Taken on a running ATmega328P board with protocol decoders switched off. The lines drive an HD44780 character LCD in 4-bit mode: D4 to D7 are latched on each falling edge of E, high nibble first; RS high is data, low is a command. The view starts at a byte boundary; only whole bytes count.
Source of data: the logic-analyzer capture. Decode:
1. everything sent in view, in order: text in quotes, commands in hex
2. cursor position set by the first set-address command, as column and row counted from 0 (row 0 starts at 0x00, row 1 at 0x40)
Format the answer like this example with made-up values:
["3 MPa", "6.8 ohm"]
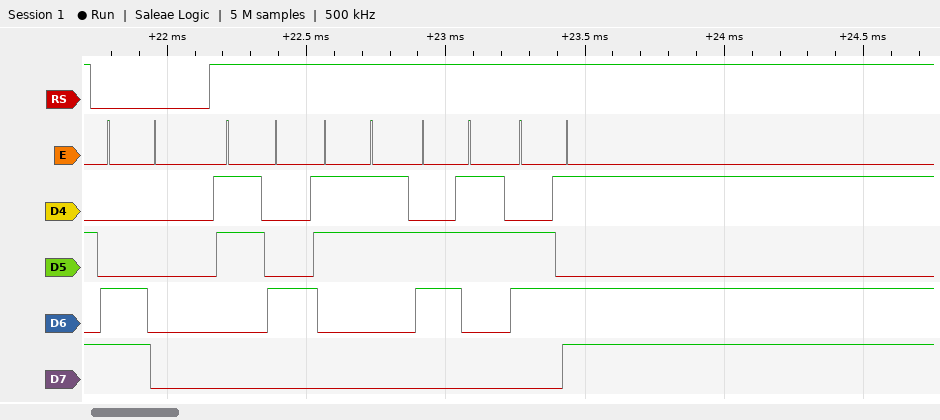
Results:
["0xC0 \"43cm\"", "column 0, row 1"]
